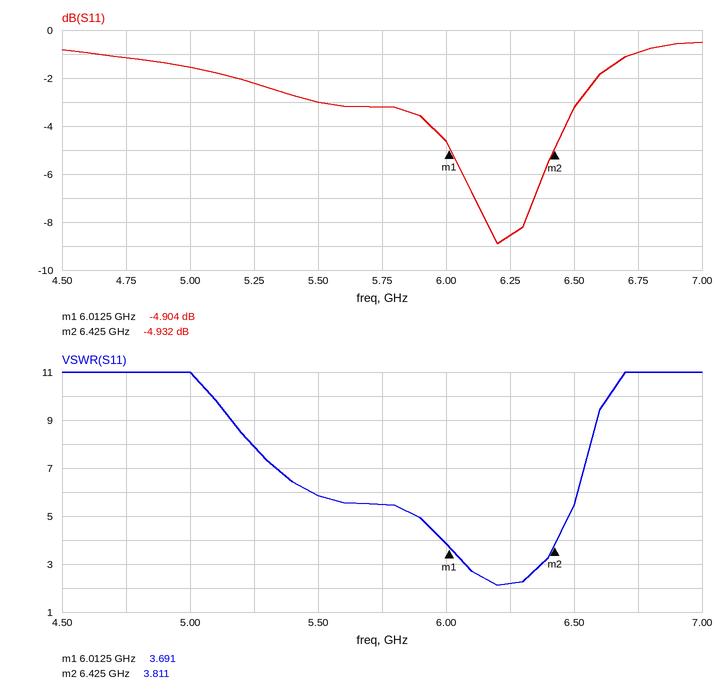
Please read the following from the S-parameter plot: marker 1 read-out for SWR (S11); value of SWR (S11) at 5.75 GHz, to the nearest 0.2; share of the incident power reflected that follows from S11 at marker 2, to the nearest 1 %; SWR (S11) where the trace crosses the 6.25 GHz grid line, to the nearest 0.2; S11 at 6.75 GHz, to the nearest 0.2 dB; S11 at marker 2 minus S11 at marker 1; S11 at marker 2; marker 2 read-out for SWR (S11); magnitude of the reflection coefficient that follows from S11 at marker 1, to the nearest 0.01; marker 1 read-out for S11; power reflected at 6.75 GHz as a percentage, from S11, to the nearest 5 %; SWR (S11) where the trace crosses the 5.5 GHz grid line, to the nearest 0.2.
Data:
3.691
5.4
32 %
2.2
-1.0 dB
-0.028 dB
-4.932 dB
3.811
0.57
-4.904 dB
80 %
5.8
